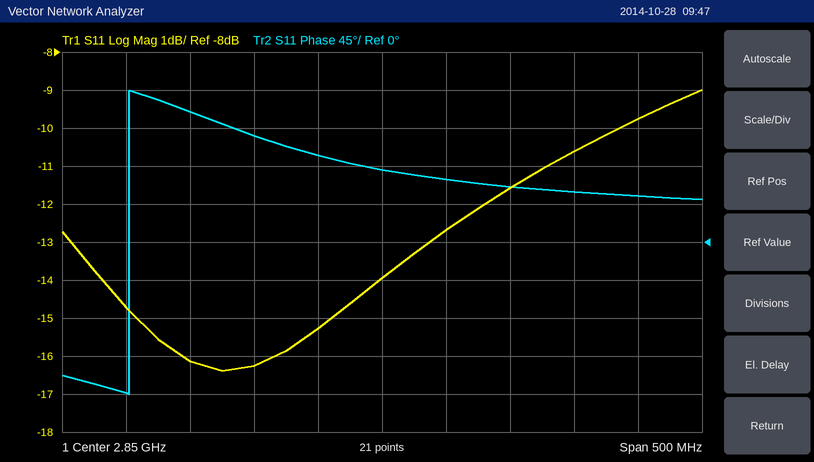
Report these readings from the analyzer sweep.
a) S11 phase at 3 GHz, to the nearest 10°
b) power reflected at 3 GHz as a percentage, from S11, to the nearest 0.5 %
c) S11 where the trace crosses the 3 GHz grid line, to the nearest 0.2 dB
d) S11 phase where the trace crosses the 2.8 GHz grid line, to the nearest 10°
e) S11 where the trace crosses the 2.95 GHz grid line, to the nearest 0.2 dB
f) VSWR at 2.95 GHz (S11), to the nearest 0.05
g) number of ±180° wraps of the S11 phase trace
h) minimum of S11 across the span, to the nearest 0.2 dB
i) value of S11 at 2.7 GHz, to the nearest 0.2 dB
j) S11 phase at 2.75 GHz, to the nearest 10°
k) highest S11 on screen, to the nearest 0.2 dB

60°
8.5 %
-10.6 dB
100°
-11.6 dB
1.70
1
-16.4 dB
-16.2 dB
130°
-9.0 dB
